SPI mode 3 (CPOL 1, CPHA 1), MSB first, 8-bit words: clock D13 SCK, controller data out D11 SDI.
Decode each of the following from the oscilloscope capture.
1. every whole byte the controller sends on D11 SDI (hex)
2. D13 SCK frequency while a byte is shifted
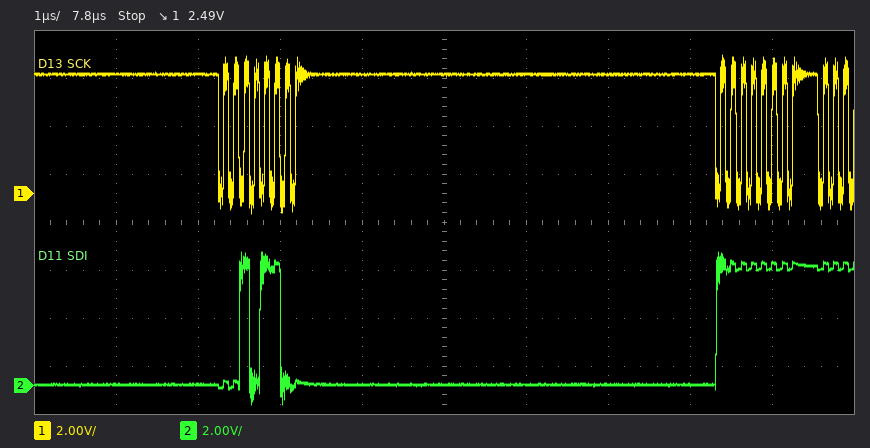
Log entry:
2C FF
8 MHz
